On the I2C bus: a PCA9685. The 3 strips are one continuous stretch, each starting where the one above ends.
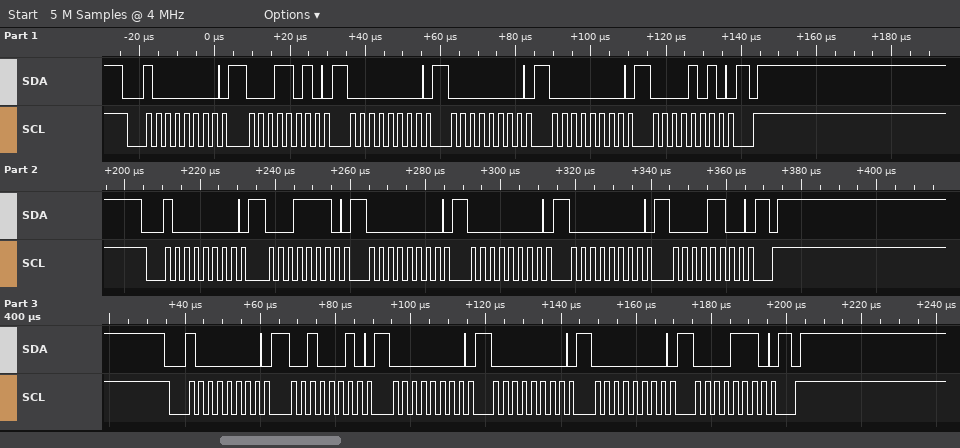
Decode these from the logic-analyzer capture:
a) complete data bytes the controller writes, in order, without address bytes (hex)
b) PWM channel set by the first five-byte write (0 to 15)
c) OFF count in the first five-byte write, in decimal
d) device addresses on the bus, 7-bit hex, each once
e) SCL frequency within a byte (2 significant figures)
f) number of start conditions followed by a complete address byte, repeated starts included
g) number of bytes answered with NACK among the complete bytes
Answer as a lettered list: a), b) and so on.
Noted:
a) 1A 00 00 00 0A 1E 00 00 00 0C 22 00 00 00 0E
b) 5
c) 2560
d) 0x40
e) 400 kHz
f) 3
g) 0
